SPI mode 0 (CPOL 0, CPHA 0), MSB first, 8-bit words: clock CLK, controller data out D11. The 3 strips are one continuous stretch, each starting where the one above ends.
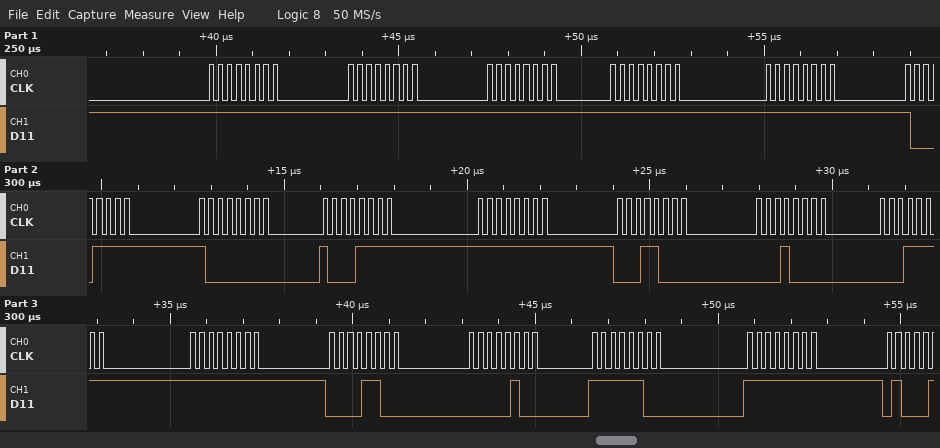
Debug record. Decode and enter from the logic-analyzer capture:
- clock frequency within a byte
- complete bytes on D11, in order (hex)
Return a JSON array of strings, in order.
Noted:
["4 MHz", "FF FF FF FF FF 8F 80 8F FF 18 10 1F FF 0C 04 FC FF"]
